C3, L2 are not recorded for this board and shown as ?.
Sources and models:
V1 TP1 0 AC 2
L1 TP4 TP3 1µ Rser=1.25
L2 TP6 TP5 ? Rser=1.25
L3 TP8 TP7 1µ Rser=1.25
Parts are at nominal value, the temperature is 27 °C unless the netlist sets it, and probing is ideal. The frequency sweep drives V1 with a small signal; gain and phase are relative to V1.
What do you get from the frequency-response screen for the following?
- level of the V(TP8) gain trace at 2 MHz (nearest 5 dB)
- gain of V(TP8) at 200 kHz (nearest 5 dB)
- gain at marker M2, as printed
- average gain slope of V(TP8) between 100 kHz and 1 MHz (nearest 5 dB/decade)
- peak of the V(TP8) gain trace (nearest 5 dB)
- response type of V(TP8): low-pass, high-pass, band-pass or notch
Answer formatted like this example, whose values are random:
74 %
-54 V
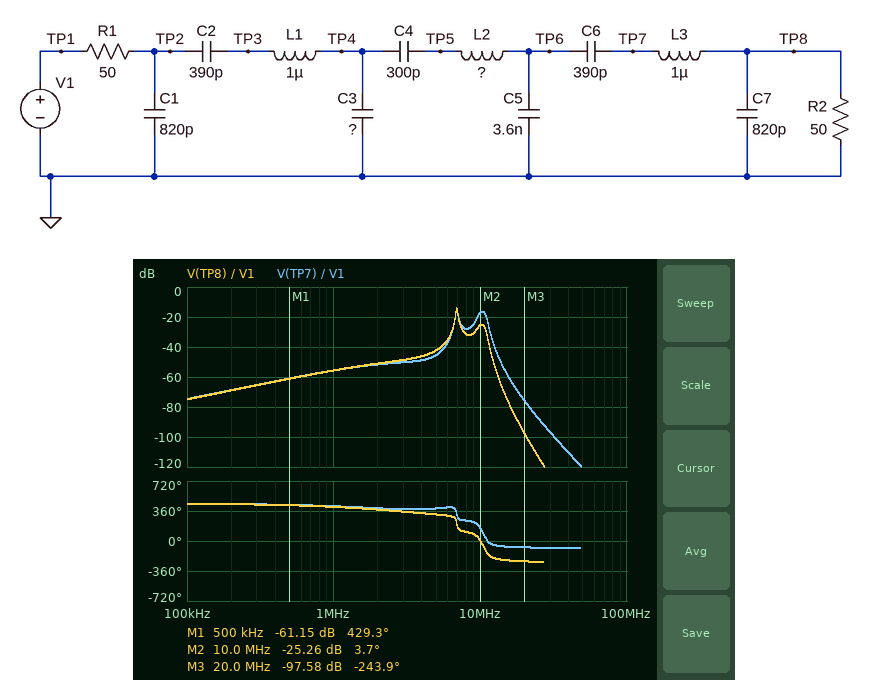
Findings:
-50 dB
-70 dB
-25.26 dB
20 dB/decade
-15 dB
band-pass
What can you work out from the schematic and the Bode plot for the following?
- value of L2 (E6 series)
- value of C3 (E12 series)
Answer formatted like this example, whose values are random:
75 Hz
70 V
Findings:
2.2 µH
1.2 nF
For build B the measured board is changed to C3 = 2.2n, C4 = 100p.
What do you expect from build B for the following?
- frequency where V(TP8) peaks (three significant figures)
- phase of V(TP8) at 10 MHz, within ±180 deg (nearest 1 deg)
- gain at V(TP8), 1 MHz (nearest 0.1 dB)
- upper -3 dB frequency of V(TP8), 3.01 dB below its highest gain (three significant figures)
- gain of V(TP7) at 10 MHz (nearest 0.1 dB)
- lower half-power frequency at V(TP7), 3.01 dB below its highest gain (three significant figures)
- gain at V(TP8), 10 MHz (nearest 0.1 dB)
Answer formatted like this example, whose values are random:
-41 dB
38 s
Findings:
11.2 MHz
124 deg
-68.0 dB
11.3 MHz
-11.7 dB
11.1 MHz
-19.9 dB
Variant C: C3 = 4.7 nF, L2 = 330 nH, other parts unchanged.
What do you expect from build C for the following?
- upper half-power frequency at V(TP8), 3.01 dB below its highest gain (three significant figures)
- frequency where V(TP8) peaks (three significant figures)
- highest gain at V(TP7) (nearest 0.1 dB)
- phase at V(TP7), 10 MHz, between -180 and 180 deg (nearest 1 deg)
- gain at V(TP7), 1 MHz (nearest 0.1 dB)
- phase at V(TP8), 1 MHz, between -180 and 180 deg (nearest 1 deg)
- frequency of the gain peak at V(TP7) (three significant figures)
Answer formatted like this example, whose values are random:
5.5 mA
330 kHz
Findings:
10.3 MHz
9.89 MHz
-20.1 dB
-104 deg
-65.0 dB
49 deg
9.94 MHz
